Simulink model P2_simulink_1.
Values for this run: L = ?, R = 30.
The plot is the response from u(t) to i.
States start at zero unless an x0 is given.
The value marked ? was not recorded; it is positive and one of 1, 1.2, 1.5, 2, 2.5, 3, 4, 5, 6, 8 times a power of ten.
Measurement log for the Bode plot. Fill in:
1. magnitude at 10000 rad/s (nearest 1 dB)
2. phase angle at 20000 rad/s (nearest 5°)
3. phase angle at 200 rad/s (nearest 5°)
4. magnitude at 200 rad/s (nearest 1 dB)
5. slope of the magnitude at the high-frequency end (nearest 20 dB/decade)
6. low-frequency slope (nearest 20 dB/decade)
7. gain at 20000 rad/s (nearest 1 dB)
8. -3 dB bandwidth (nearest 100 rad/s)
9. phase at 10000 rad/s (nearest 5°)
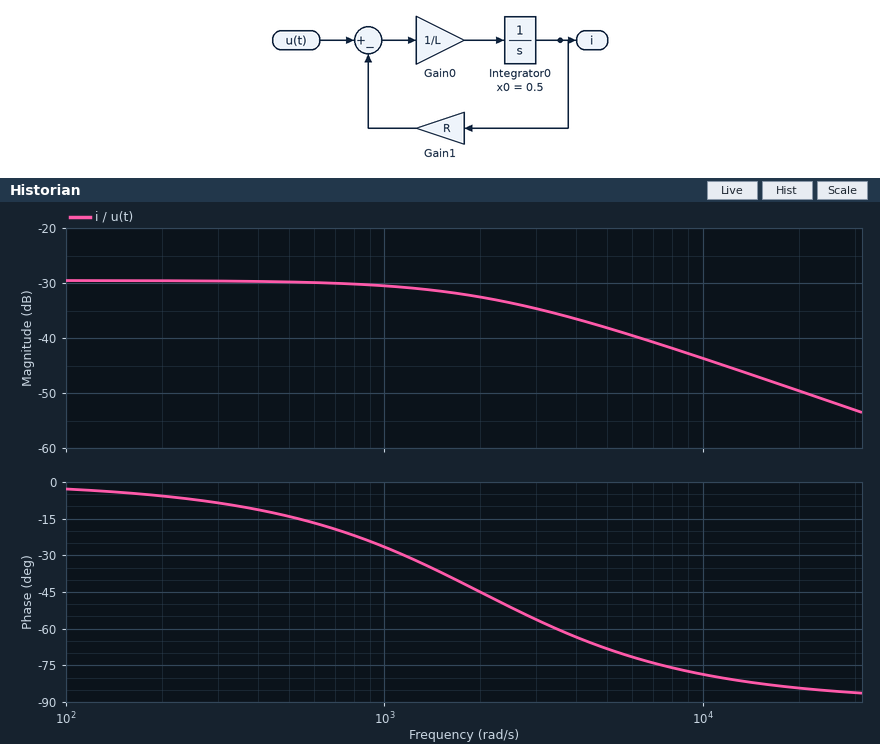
-44 dB
-85°
-5°
-30 dB
-20 dB/decade
0 dB/decade
-50 dB
2000 rad/s
-80°
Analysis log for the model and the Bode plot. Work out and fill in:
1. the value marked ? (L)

0.015
